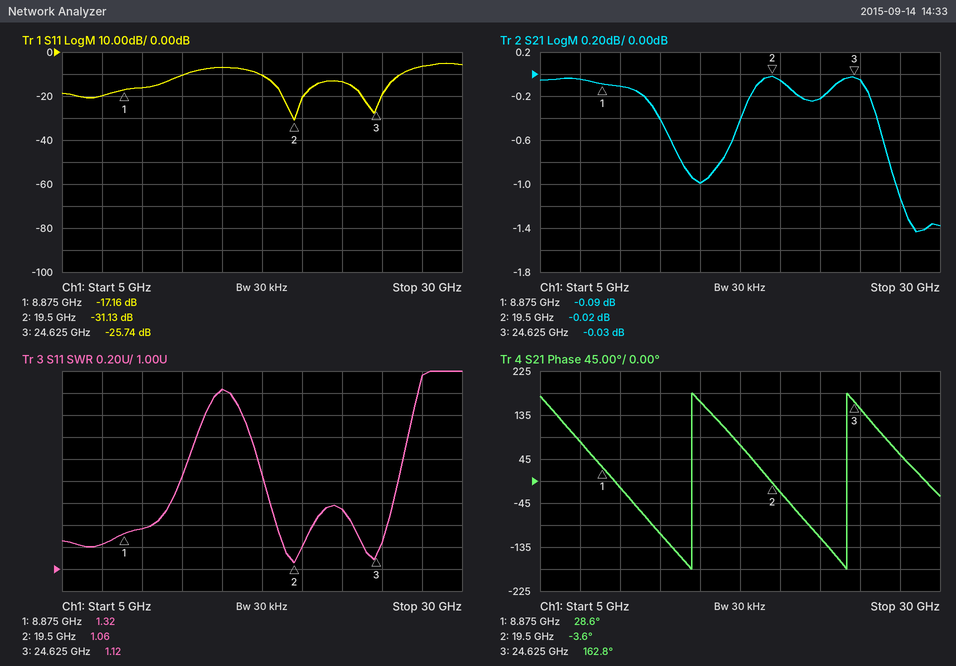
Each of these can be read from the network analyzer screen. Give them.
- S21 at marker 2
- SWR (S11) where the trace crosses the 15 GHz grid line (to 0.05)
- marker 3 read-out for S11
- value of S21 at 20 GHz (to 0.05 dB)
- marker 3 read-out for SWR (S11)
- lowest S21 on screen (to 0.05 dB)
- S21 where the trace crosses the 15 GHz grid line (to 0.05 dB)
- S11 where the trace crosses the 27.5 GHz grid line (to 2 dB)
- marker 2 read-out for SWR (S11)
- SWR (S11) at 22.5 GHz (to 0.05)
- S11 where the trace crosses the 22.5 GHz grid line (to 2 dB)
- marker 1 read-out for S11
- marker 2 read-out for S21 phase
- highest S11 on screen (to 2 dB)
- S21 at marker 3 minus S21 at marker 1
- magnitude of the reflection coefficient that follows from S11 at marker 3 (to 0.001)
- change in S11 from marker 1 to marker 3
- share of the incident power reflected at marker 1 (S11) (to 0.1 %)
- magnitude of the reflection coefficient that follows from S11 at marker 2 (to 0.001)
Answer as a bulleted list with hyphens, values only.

- -0.02 dB
- 2.65
- -25.74 dB
- -0.05 dB
- 1.12
- -1.45 dB
- -1.00 dB
- -6 dB
- 1.06
- 1.55
- -14 dB
- -17.16 dB
- -3.6°
- -6 dB
- 0.06 dB
- 0.052
- -8.58 dB
- 1.9 %
- 0.028
